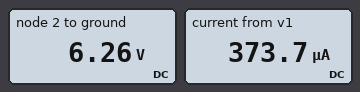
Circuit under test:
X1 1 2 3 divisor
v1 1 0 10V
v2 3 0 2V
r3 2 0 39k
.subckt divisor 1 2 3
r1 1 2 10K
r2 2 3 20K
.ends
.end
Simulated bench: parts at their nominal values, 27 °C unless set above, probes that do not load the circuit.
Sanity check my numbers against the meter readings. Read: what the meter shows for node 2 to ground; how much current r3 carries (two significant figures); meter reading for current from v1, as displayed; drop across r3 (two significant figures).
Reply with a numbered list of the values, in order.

1. 6.26 V
2. 160 µA
3. 373.7 µA
4. 6.3 V
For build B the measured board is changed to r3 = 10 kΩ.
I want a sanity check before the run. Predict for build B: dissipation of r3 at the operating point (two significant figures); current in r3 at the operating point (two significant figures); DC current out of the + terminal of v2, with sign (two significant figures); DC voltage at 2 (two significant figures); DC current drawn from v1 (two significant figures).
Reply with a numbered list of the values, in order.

1. 1.9 mW
2. 440 µA
3. -120 µA
4. 4.4 V
5. 560 µA
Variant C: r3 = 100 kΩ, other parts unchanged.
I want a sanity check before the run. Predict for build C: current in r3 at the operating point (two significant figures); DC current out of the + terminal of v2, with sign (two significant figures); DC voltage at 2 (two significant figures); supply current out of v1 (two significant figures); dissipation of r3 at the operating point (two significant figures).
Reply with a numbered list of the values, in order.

1. 69 µA
2. -240 µA
3. 6.9 V
4. 310 µA
5. 470 µW
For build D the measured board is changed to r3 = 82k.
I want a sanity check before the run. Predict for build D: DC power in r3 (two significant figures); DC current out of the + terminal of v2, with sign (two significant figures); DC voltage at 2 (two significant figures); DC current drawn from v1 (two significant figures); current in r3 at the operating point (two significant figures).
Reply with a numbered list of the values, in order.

1. 560 µW
2. -240 µA
3. 6.8 V
4. 320 µA
5. 83 µA
